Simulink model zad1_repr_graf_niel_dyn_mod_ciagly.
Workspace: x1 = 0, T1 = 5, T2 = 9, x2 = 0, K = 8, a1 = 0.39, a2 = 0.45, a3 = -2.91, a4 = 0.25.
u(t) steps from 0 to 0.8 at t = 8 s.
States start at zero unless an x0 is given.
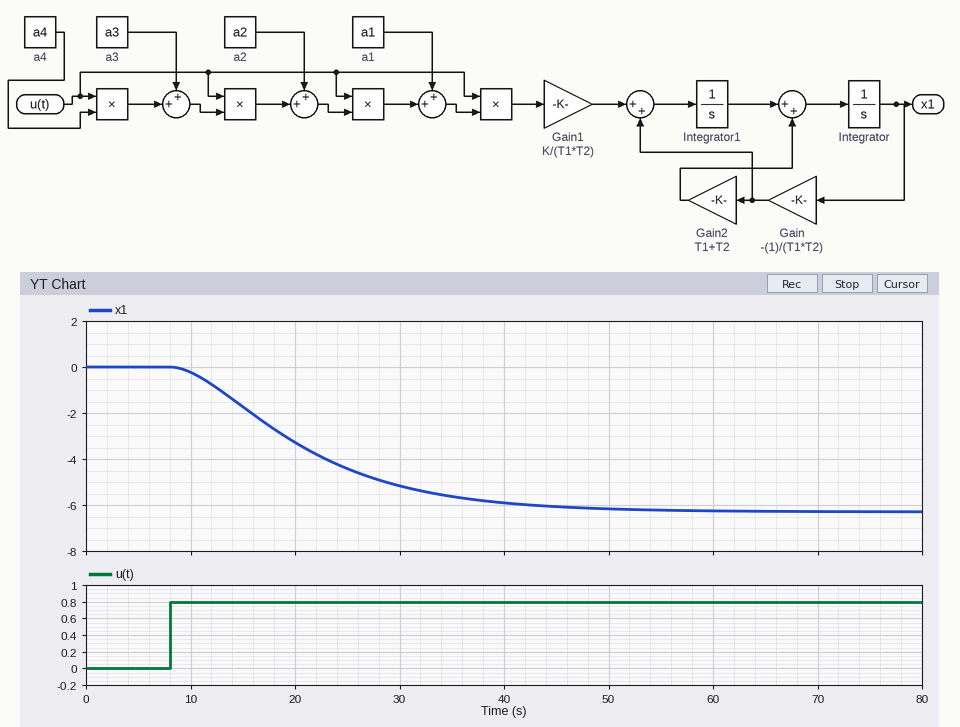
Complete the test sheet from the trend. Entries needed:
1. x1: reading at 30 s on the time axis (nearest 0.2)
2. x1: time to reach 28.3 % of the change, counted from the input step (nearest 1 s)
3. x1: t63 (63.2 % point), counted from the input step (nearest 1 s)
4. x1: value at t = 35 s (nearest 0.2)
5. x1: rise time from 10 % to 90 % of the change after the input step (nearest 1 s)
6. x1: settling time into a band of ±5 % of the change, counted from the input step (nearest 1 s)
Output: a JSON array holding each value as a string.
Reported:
["-5.2", "7 s", "15 s", "-5.6", "24 s", "34 s"]
